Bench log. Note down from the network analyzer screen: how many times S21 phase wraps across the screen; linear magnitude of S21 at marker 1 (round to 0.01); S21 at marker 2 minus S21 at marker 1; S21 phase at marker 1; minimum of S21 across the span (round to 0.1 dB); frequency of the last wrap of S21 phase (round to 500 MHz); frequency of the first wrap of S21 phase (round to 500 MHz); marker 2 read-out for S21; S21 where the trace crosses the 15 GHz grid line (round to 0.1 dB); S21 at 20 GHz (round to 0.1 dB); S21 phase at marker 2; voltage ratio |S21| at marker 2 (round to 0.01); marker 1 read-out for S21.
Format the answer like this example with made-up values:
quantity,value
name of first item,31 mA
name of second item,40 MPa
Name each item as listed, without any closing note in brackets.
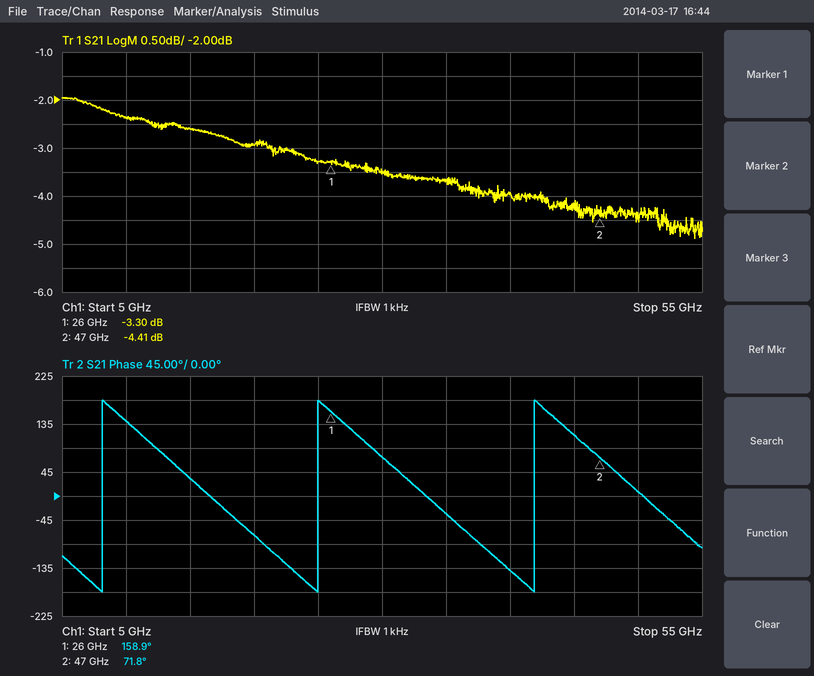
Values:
quantity,value
how many times S21 phase wraps across the screen,3
linear magnitude of S21 at marker 1,0.68
S21 at marker 2 minus S21 at marker 1,-1.11 dB
S21 phase at marker 1,158.9°
minimum of S21 across the span,-4.9 dB
frequency of the last wrap of S21 phase,42.0 GHz
frequency of the first wrap of S21 phase,8.0 GHz
marker 2 read-out for S21,-4.41 dB
S21 where the trace crosses the 15 GHz grid line,-2.6 dB
S21 at 20 GHz,-2.9 dB
S21 phase at marker 2,71.8°
voltage ratio |S21| at marker 2,0.60
marker 1 read-out for S21,-3.30 dB
